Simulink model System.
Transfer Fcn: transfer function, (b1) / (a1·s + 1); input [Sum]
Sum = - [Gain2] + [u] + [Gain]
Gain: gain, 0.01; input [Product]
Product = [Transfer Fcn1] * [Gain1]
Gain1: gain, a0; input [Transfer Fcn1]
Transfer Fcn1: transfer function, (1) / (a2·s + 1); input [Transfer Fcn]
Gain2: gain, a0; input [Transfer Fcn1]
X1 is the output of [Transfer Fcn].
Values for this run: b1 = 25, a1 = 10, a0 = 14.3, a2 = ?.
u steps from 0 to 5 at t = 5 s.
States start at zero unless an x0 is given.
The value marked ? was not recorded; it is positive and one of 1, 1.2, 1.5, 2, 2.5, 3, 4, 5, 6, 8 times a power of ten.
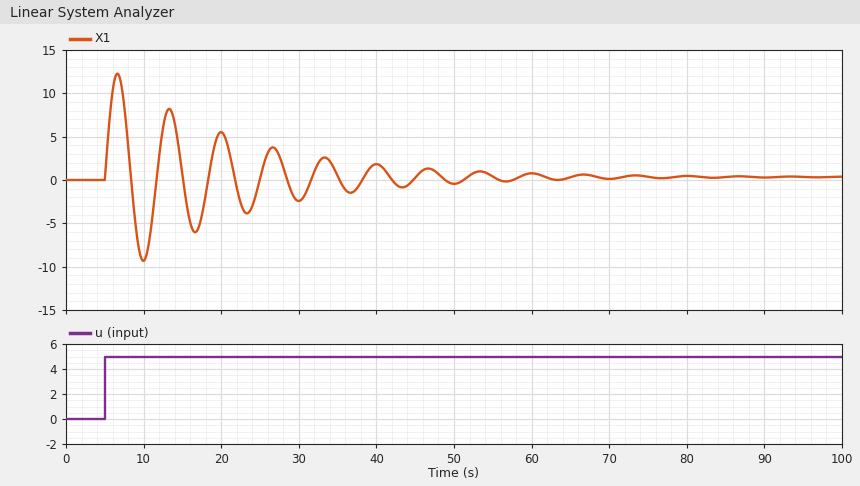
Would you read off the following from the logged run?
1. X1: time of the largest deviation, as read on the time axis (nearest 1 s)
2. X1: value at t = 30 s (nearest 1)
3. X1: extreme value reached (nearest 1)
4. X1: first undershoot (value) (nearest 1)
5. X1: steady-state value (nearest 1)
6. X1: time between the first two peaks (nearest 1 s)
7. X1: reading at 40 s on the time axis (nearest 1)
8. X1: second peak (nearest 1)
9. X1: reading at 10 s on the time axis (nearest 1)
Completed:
7 s
-2
12
-9
0
7 s
2
8
-9
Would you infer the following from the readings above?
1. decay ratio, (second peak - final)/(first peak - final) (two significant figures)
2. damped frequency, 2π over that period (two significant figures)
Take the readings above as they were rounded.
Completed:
0.67
0.90 rad/s
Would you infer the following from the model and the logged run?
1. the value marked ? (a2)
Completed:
40
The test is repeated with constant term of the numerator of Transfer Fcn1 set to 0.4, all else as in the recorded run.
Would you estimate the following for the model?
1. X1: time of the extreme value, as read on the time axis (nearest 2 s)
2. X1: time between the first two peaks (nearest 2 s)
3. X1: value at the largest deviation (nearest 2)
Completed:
8 s
10 s
18
